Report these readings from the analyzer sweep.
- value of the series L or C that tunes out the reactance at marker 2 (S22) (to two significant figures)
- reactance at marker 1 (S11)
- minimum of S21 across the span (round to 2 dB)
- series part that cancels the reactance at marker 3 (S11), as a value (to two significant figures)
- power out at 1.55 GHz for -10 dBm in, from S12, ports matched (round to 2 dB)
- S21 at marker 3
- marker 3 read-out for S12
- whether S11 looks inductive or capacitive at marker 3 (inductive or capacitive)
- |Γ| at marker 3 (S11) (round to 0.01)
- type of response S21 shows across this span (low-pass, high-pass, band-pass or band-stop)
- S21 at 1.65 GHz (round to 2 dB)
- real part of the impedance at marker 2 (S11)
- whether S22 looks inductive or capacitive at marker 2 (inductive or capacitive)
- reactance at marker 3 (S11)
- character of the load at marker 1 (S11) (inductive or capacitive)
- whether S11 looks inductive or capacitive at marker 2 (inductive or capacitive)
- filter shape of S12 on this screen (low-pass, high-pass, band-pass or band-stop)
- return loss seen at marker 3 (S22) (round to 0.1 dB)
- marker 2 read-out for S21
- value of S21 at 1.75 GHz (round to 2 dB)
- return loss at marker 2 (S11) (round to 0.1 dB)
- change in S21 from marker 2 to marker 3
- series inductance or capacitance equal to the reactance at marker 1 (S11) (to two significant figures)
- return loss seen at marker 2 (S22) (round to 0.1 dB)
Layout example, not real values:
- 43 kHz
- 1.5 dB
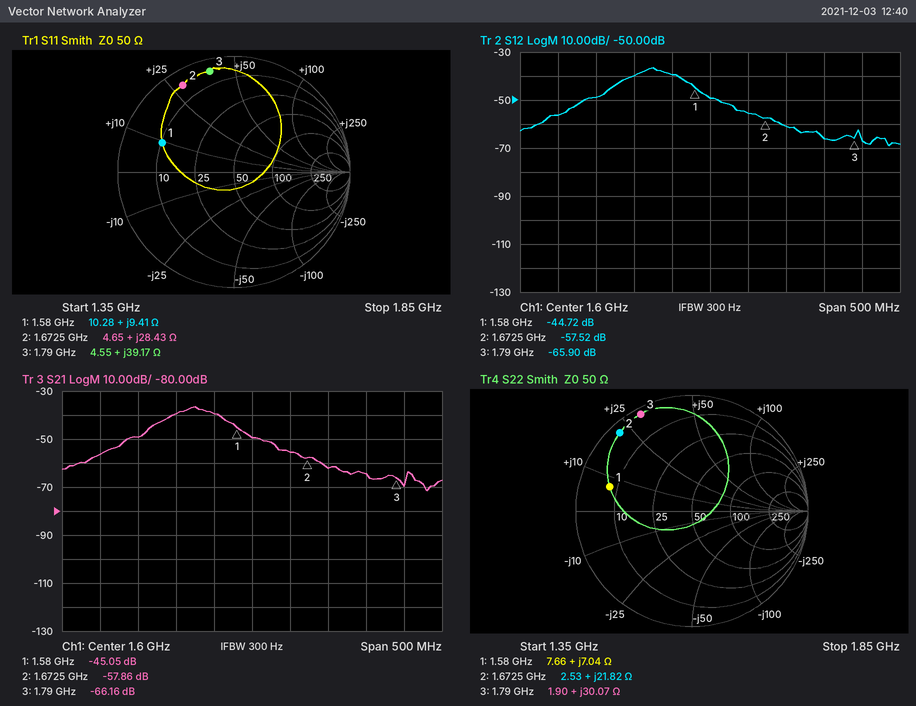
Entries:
- 4.4 pF
- +9.41 Ω
- -72 dB
- 2.3 pF
- -50 dBm
- -66.16 dB
- -65.90 dB
- inductive
- 0.89
- band-pass
- -56 dB
- 4.65 Ω
- inductive
- +39.17 Ω
- inductive
- inductive
- band-pass
- 0.5 dB
- -57.86 dB
- -64 dB
- 1.2 dB
- -8.30 dB
- 950 pH
- 0.7 dB
